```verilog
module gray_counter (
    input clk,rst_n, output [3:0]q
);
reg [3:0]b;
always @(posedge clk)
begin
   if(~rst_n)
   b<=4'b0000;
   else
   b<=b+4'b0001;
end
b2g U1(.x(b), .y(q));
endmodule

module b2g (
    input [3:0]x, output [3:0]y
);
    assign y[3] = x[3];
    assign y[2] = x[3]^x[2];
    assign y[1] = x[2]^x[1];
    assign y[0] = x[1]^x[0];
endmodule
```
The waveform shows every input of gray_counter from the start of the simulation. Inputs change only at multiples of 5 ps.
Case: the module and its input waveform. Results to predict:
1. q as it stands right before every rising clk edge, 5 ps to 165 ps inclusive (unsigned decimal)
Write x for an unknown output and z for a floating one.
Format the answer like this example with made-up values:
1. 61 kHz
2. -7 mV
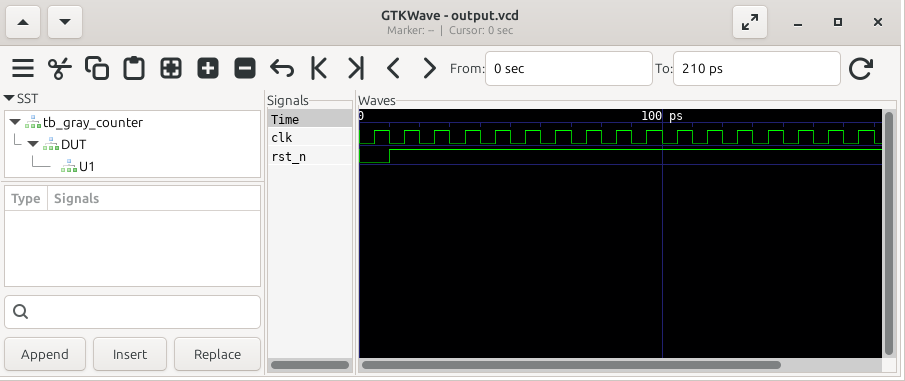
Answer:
1. x, 0, 1, 3, 2, 6, 7, 5, 4, 12, 13, 15, 14, 10, 11, 9, 8
